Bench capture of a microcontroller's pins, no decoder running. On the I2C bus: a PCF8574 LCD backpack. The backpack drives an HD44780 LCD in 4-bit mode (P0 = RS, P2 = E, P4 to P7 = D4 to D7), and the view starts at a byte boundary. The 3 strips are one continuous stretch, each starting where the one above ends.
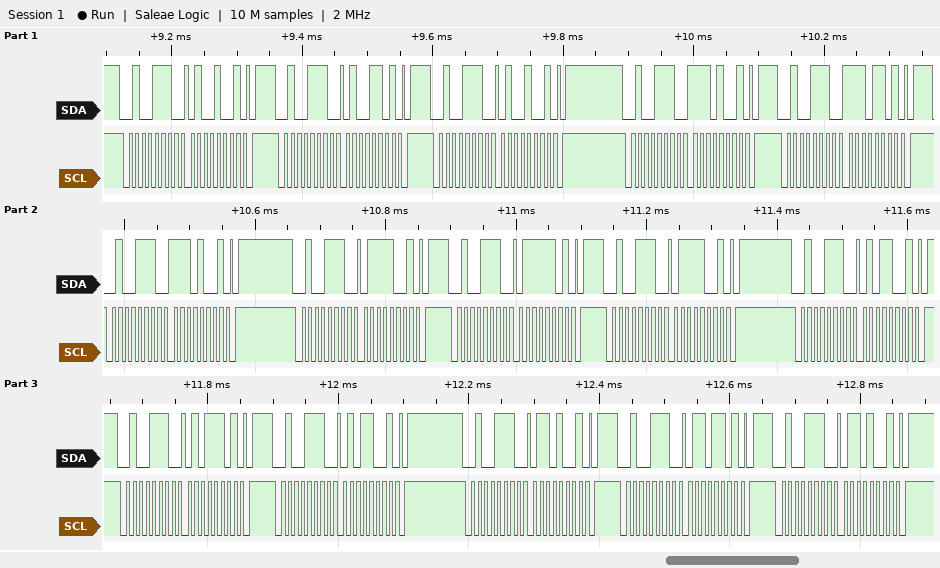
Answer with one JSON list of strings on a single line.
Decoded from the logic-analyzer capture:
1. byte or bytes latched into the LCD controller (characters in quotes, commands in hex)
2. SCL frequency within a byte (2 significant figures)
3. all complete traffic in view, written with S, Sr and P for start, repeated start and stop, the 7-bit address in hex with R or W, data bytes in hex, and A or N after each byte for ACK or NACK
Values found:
["'N' 'u'", "100 kHz", "S 27W A 49 A P S 27W A 4D A P S 27W A 49 A P S 27W A E9 A P S 27W A ED A P S 27W A E9 A P S 27W A 79 A P S 27W A 7D A P S 27W A 79 A P S 27W A 59 A P S 27W A 5D A P S 27W A 59 A P S 27W A 69 A P S 27W A 6D A P S 27W A 69 A P"]
